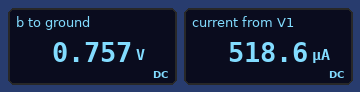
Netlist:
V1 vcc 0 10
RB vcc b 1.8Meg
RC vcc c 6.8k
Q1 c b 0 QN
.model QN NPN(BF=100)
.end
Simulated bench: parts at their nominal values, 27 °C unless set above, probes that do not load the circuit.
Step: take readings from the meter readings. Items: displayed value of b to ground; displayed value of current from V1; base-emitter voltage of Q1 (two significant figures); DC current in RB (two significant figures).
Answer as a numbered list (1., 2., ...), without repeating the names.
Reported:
1. 0.757 V
2. 518.6 µA
3. 760 mV
4. 5.1 µA
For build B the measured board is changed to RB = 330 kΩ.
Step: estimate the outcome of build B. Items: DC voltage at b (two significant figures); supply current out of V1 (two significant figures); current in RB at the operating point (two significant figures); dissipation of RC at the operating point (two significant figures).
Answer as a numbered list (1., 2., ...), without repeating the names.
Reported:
1. 780 mV
2. 1.5 mA
3. 28 µA
4. 14 mW
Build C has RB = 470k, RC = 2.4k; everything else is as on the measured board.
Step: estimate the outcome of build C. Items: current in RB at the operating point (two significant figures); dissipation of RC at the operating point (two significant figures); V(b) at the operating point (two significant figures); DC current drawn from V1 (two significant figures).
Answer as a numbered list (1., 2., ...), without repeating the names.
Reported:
1. 20 µA
2. 9.2 mW
3. 790 mV
4. 2.0 mA
